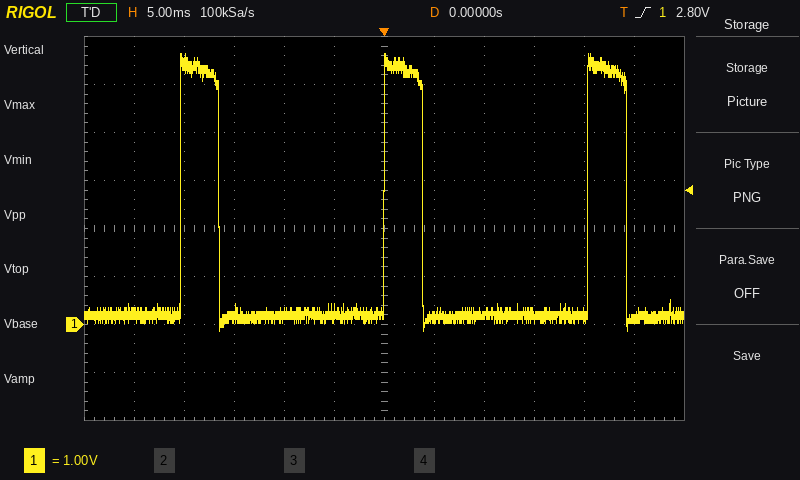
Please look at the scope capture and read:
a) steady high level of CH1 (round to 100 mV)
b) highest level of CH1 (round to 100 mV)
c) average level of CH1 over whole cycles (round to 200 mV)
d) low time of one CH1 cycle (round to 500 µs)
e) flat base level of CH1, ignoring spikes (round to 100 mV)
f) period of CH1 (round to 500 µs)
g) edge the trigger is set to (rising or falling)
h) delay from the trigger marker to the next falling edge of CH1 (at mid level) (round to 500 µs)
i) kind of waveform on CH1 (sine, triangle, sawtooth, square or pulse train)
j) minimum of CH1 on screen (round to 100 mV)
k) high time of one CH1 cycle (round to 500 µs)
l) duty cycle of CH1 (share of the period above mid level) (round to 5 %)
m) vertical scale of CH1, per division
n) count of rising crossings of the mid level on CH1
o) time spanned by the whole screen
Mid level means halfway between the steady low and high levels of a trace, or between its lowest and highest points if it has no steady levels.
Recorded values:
5.3 V
5.6 V
1.2 V
16.5 ms
200 mV
20.5 ms
rising
4.0 ms
pulse train
-100 mV
4.0 ms
20 %
1 V
3
60 ms
